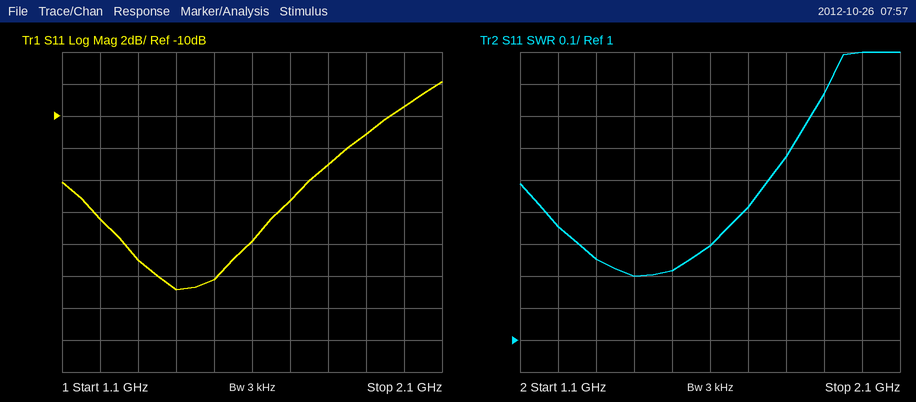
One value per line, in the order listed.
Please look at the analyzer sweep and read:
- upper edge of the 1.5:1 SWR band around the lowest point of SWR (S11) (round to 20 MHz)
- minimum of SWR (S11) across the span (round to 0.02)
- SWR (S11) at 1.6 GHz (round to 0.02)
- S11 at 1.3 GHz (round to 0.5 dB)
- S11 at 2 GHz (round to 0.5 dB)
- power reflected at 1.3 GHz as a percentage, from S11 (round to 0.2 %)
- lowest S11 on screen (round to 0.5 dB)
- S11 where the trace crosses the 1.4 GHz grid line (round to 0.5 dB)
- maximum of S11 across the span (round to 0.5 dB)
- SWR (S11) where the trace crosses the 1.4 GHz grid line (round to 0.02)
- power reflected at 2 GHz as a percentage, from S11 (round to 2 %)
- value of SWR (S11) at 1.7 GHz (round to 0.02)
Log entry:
1.76 GHz
1.20
1.30
-19.0 dB
-9.5 dB
1.2 %
-21.0 dB
-21.0 dB
-8.0 dB
1.20
12 %
1.42
